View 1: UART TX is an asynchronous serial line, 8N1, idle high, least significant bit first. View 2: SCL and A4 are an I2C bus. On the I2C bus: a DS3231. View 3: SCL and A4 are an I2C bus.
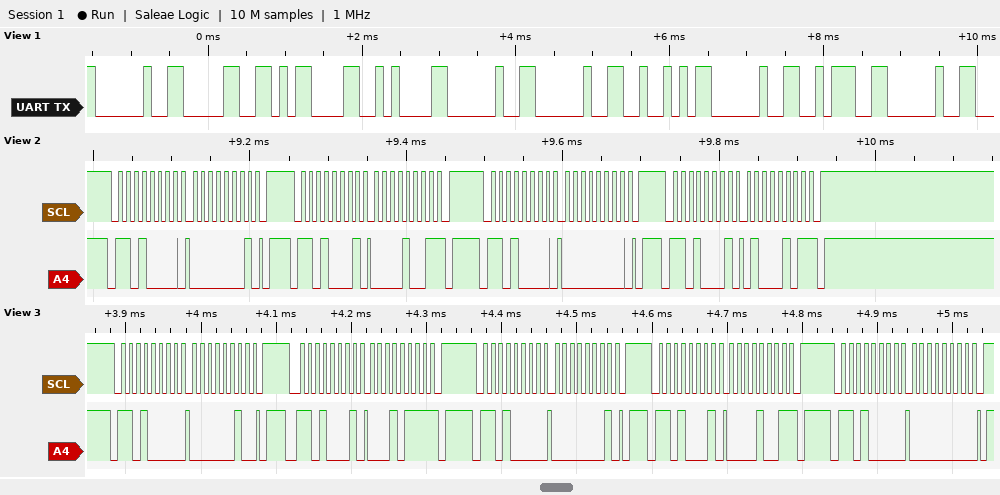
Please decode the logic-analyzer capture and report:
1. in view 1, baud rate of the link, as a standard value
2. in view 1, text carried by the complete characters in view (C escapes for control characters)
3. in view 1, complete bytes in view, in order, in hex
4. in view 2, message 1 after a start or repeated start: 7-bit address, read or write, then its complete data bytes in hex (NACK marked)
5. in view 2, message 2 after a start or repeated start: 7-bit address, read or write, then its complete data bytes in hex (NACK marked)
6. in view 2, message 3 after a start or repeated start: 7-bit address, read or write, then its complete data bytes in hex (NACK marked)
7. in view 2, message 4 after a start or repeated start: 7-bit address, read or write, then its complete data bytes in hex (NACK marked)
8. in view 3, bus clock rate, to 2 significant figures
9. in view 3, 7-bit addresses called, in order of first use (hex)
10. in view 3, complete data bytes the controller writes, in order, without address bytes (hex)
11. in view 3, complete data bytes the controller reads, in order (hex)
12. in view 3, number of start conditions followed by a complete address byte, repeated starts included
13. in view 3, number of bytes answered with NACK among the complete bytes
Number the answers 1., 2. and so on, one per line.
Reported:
1. 9600 baud
2. " 0\r\n  R : "
3. 20 30 0D 0A 20 20 52 20 3A 20
4. 0x68 write: 01
5. 0x68 read: 09 NACK
6. 0x68 write: 00
7. 0x68 read: 45 NACK
8. 100 kHz
9. 0x68
10. 02 01 00
11. 17 09
12. 5
13. 2
